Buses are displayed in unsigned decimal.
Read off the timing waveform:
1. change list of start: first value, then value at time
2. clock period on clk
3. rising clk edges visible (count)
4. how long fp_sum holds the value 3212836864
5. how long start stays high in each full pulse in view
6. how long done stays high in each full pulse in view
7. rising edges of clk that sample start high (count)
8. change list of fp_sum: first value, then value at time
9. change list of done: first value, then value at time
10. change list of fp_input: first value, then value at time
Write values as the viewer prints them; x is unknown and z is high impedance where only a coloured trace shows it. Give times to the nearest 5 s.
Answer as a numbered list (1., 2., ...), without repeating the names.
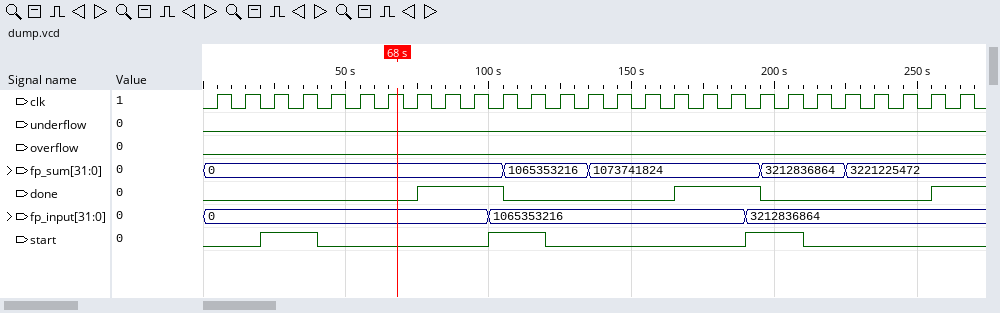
1. 0, 1 at 20 s, 0 at 40 s, 1 at 100 s, 0 at 120 s, 1 at 190 s, 0 at 210 s
2. 10 s
3. 27
4. 30 s
5. 20 s, 20 s, 20 s
6. 30 s, 30 s
7. 6
8. 0, 1065353216 at 105 s, 1073741824 at 135 s, 3212836864 at 195 s, 3221225472 at 225 s
9. 0, 1 at 75 s, 0 at 105 s, 1 at 165 s, 0 at 195 s, 1 at 255 s
10. 0, 1065353216 at 100 s, 3212836864 at 190 s
